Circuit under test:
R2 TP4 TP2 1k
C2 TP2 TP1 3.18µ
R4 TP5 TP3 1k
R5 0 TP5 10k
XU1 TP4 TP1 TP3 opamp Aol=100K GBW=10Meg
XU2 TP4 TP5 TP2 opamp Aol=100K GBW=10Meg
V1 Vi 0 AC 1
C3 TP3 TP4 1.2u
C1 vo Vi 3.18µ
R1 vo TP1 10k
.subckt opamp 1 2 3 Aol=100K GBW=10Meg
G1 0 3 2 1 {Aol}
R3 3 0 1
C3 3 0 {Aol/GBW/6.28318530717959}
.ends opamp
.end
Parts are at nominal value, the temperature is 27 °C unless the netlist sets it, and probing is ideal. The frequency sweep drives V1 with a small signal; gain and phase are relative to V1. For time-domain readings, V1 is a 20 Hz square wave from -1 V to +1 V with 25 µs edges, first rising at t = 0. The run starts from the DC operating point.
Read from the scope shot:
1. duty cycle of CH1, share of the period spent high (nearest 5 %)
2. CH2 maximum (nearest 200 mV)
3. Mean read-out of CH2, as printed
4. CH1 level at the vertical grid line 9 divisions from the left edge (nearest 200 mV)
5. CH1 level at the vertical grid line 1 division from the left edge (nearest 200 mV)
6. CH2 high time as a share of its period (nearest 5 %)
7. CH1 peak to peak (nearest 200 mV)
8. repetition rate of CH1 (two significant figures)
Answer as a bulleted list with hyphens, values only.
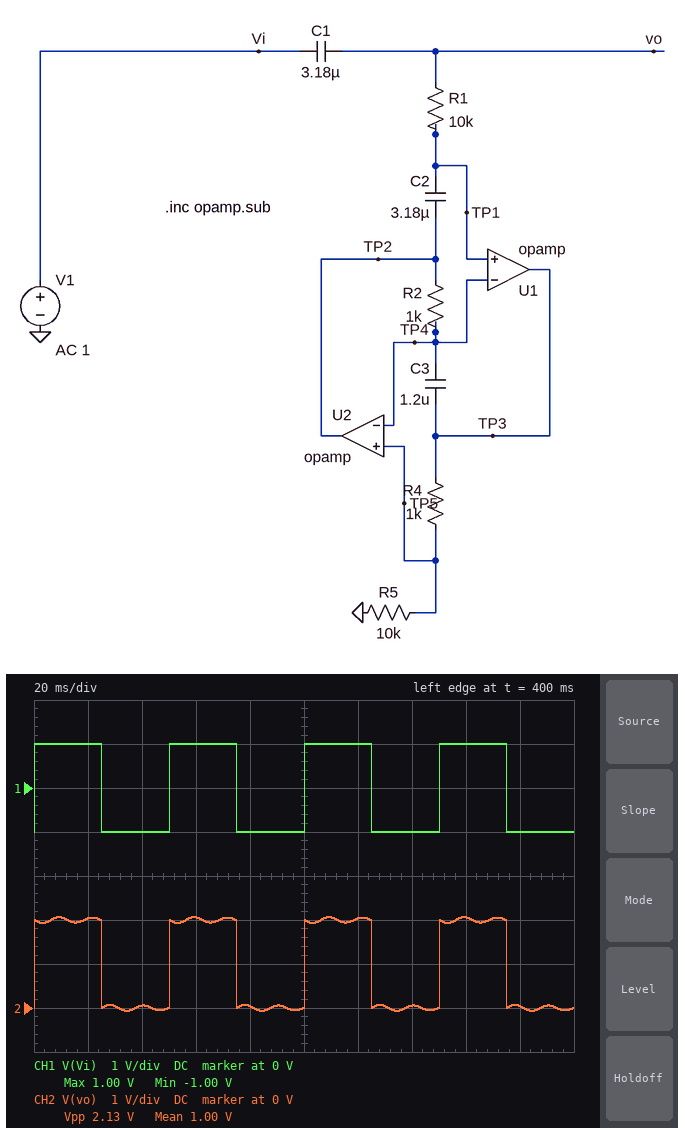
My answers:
- 50 %
- 2.0 V
- 1.00 V
- -1.0 V
- 1.0 V
- 50 %
- 2.0 V
- 20 Hz
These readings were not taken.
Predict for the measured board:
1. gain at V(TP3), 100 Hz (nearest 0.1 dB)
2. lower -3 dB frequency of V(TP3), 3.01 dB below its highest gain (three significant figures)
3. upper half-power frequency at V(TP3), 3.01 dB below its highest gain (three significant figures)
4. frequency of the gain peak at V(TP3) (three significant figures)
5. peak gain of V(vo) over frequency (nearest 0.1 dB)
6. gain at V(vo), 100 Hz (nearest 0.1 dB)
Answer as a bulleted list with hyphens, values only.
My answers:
- 6.6 dB
- 78.8 Hz
- 83.9 Hz
- 81.4 Hz
- 0 dB
- -0.1 dB
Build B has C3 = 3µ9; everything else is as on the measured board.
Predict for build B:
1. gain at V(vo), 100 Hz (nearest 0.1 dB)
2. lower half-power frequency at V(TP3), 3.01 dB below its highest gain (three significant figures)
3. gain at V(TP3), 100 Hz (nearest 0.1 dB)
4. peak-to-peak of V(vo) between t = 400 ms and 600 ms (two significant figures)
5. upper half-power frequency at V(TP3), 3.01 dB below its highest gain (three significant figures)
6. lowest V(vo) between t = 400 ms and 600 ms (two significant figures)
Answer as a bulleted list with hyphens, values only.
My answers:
- 0 dB
- 42.5 Hz
- -11.0 dB
- 2.2 V
- 47.5 Hz
- -110 mV
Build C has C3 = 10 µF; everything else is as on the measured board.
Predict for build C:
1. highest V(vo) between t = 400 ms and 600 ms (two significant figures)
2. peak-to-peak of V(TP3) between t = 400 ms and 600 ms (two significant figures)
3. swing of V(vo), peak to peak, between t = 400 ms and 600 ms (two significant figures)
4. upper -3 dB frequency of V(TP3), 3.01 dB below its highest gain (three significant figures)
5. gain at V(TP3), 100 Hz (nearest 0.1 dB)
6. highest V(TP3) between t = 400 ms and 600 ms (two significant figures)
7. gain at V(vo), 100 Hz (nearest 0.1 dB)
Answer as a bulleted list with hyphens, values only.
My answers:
- 2.2 V
- 5.6 V
- 2.5 V
- 30.4 Hz
- -20.4 dB
- 3.9 V
- 0 dB
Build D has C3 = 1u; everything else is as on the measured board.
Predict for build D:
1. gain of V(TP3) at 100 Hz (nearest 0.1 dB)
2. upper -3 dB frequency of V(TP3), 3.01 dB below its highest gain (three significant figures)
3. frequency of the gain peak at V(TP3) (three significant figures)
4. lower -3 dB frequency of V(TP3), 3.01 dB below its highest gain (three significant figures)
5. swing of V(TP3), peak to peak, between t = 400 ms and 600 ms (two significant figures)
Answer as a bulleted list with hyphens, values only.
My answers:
- 12.4 dB
- 91.6 Hz
- 89.2 Hz
- 86.6 Hz
- 5.3 V
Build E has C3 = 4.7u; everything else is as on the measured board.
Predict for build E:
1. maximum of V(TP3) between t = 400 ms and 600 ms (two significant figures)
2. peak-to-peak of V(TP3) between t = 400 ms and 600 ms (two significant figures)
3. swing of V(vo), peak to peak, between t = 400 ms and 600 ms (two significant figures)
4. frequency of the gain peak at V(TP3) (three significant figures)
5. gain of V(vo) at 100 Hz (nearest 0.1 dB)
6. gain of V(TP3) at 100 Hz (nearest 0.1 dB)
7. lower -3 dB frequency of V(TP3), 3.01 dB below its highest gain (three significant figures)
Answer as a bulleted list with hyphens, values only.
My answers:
- 3.3 V
- 4.4 V
- 2.2 V
- 41.0 Hz
- 0 dB
- -13.0 dB
- 38.4 Hz
